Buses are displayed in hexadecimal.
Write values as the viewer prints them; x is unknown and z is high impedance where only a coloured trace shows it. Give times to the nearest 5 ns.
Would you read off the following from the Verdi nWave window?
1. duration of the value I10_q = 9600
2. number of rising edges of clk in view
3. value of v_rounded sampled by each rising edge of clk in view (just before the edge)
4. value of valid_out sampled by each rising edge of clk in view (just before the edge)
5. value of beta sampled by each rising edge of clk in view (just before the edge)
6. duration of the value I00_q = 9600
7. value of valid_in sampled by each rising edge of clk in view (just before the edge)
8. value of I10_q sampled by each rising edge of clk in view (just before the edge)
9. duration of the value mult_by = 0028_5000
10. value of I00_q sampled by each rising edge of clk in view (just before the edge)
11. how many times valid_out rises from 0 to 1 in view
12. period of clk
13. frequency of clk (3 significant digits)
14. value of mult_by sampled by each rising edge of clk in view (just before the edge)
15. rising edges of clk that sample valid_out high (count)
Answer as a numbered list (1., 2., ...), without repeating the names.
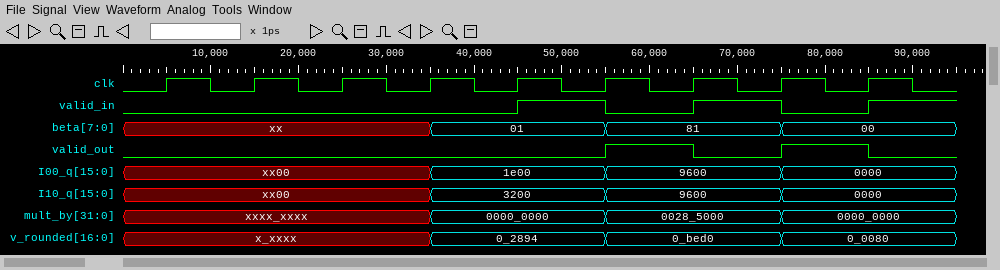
1. 20 ns
2. 9
3. x_xxxx, x_xxxx, x_xxxx, x_xxxx, 0_2894, 0_2894, 0_bed0, 0_bed0, 0_0080
4. 0 0 0 0 0 0 1 0 1
5. xx, xx, xx, xx, 01, 01, 81, 81, 00
6. 20 ns
7. 0 0 0 0 0 1 0 1 0
8. xx00, xx00, xx00, xx00, 3200, 3200, 9600, 9600, 0000
9. 20 ns
10. xx00, xx00, xx00, xx00, 1e00, 1e00, 9600, 9600, 0000
11. 2
12. 10 ns
13. 100 MHz
14. xxxx_xxxx, xxxx_xxxx, xxxx_xxxx, xxxx_xxxx, 0000_0000, 0000_0000, 0028_5000, 0028_5000, 0000_0000
15. 2
